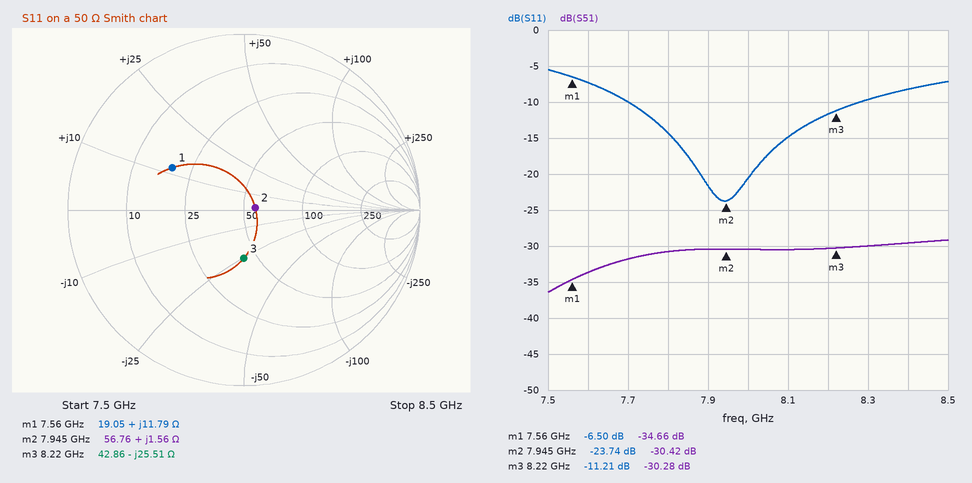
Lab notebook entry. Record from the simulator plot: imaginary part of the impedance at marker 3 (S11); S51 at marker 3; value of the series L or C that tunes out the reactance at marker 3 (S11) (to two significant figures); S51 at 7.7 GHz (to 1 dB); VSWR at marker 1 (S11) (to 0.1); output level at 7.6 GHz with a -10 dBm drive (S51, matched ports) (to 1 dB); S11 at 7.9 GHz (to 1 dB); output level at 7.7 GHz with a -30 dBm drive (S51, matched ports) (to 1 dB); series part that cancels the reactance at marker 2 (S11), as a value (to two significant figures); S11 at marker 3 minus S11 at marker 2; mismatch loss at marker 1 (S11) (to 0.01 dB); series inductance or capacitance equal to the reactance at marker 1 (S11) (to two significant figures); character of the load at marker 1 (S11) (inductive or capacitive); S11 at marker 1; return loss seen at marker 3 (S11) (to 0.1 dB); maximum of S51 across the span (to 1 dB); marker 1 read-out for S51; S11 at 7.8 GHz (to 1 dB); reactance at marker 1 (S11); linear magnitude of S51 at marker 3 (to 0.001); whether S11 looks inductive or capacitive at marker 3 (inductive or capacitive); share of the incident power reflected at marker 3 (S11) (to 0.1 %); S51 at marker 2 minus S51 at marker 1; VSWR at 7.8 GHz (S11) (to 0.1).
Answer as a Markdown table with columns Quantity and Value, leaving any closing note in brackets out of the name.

| Quantity | Value |
|---|---|
| imaginary part of the impedance at marker 3 | -25.51 Ω |
| S51 at marker 3 | -30.28 dB |
| value of the series L or C that tunes out the reactance at marker 3 (S11) | 490 pH |
| S51 at 7.7 GHz | -32 dB |
| VSWR at marker 1 (S11) | 2.8 |
| output level at 7.6 GHz with a -10 dBm drive (S51, matched ports) | -44 dBm |
| S11 at 7.9 GHz | -22 dB |
| output level at 7.7 GHz with a -30 dBm drive (S51, matched ports) | -62 dBm |
| series part that cancels the reactance at marker 2 (S11), as a value | 13 pF |
| S11 at marker 3 minus S11 at marker 2 | 12.53 dB |
| mismatch loss at marker 1 (S11) | 1.10 dB |
| series inductance or capacitance equal to the reactance at marker 1 (S11) | 250 pH |
| character of the load at marker 1 (S11) | inductive |
| S11 at marker 1 | -6.50 dB |
| return loss seen at marker 3 (S11) | 11.2 dB |
| maximum of S51 across the span | -29 dB |
| marker 1 read-out for S51 | -34.66 dB |
| S11 at 7.8 GHz | -14 dB |
| reactance at marker 1 | +11.79 Ω |
| linear magnitude of S51 at marker 3 | 0.031 |
| whether S11 looks inductive or capacitive at marker 3 | capacitive |
| share of the incident power reflected at marker 3 (S11) | 7.6 % |
| S51 at marker 2 minus S51 at marker 1 | 4.24 dB |
| VSWR at 7.8 GHz (S11) | 1.5 |
